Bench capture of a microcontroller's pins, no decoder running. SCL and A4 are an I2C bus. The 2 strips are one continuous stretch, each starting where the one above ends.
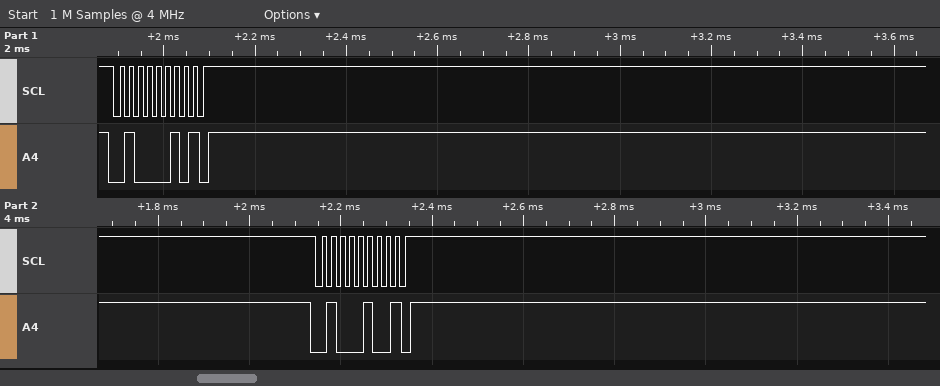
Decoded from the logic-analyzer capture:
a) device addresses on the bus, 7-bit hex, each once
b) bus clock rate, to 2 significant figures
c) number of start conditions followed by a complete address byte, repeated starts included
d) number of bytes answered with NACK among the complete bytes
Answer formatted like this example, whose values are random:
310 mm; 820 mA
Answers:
0x21 0x22; 50 kHz; 2; 2
